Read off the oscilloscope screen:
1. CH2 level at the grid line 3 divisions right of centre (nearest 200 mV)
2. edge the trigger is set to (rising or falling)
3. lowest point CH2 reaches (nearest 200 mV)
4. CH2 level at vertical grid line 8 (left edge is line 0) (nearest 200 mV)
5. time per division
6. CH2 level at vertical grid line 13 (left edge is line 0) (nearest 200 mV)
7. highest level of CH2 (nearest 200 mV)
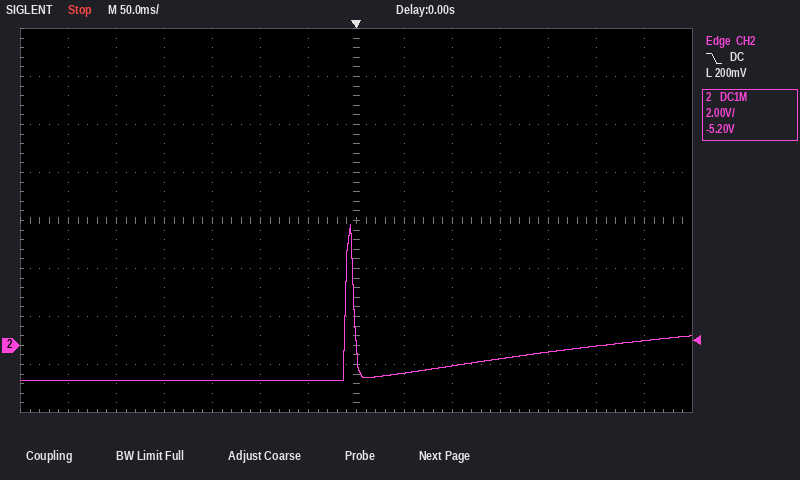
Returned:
-600 mV
falling
-1.4 V
-1.2 V
50 ms
200 mV
5.0 V
